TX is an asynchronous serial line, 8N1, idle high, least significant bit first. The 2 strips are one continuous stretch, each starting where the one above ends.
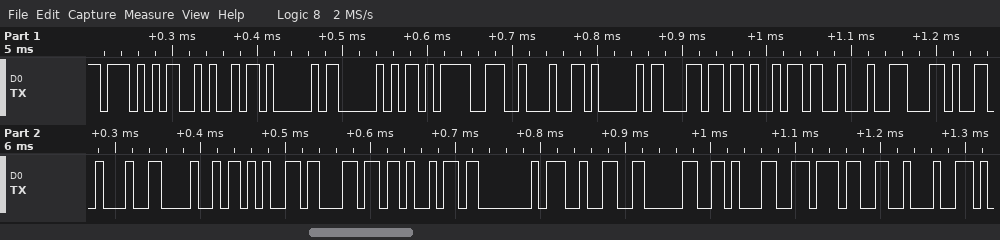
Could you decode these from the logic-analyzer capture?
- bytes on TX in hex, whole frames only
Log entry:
57 4A 41 50 3D 22 41 6C 69 22 2C 22 48 65 6C 69 40 32 30 31 37 22
